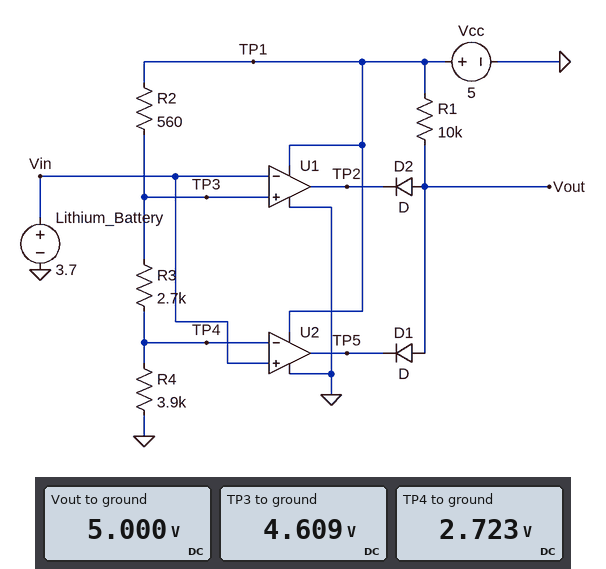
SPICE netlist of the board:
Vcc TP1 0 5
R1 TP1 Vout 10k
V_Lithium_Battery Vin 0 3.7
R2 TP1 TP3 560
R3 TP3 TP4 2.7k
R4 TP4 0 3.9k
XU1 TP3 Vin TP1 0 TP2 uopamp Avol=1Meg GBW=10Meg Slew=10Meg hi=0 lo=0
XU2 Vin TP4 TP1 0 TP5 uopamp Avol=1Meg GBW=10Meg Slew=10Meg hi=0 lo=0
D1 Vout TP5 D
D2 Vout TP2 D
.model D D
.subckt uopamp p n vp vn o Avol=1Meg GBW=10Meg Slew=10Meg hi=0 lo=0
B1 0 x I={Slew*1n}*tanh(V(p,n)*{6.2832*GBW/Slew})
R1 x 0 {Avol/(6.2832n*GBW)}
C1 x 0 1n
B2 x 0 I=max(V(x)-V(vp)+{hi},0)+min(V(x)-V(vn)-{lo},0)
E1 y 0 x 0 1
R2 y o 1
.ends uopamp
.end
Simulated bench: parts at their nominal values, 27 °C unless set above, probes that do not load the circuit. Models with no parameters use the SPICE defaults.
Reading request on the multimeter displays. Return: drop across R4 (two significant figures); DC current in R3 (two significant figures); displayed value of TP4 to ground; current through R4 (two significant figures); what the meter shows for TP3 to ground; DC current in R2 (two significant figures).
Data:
2.7 V
700 µA
2.723 V
700 µA
4.609 V
700 µA
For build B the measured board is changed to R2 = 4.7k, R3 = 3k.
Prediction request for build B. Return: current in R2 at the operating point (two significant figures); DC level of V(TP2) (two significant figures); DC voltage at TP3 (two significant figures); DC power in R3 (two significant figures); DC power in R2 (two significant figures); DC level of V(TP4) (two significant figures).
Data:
430 µA
-9.6 mV
3.0 V
560 µW
870 µW
1.7 V
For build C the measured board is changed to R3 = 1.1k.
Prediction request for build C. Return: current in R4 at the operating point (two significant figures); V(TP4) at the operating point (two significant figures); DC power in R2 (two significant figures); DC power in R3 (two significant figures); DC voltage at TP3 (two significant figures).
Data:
900 µA
3.5 V
450 µW
890 µW
4.5 V
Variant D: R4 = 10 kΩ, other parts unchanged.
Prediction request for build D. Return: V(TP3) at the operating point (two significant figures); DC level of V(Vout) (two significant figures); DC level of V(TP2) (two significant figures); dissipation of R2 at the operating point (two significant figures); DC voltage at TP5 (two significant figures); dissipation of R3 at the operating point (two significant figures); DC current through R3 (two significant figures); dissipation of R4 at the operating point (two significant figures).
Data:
4.8 V
630 mV
5.0 V
80 µW
-3.7 mV
380 µW
380 µA
1.4 mW
